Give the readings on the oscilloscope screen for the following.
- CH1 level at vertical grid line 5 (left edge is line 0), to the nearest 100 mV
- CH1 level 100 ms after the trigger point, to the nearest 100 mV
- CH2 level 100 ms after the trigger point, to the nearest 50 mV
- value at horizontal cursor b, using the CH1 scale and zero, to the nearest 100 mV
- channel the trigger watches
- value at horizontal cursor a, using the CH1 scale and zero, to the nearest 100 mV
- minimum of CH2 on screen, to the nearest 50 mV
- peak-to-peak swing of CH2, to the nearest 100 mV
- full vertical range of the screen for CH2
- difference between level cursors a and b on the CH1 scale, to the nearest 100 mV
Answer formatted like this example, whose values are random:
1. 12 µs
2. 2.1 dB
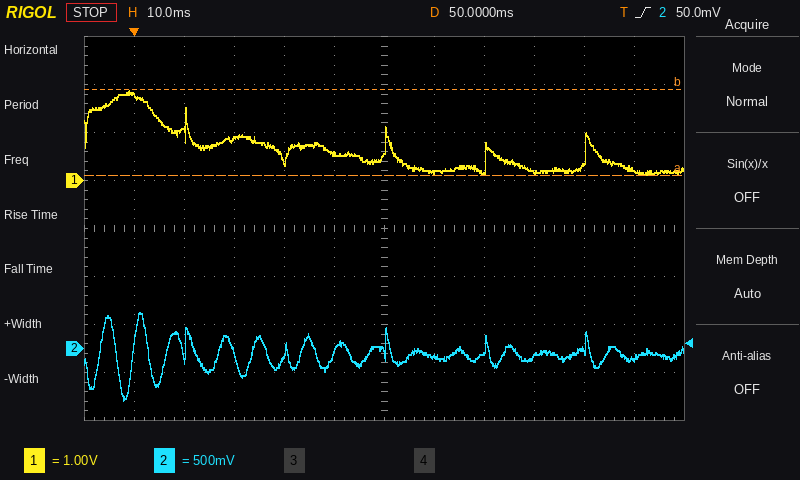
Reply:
1. 600 mV
2. 200 mV
3. -100 mV
4. 1.9 V
5. CH2
6. 100 mV
7. -550 mV
8. 900 mV
9. 4 V
10. 1.8 V
